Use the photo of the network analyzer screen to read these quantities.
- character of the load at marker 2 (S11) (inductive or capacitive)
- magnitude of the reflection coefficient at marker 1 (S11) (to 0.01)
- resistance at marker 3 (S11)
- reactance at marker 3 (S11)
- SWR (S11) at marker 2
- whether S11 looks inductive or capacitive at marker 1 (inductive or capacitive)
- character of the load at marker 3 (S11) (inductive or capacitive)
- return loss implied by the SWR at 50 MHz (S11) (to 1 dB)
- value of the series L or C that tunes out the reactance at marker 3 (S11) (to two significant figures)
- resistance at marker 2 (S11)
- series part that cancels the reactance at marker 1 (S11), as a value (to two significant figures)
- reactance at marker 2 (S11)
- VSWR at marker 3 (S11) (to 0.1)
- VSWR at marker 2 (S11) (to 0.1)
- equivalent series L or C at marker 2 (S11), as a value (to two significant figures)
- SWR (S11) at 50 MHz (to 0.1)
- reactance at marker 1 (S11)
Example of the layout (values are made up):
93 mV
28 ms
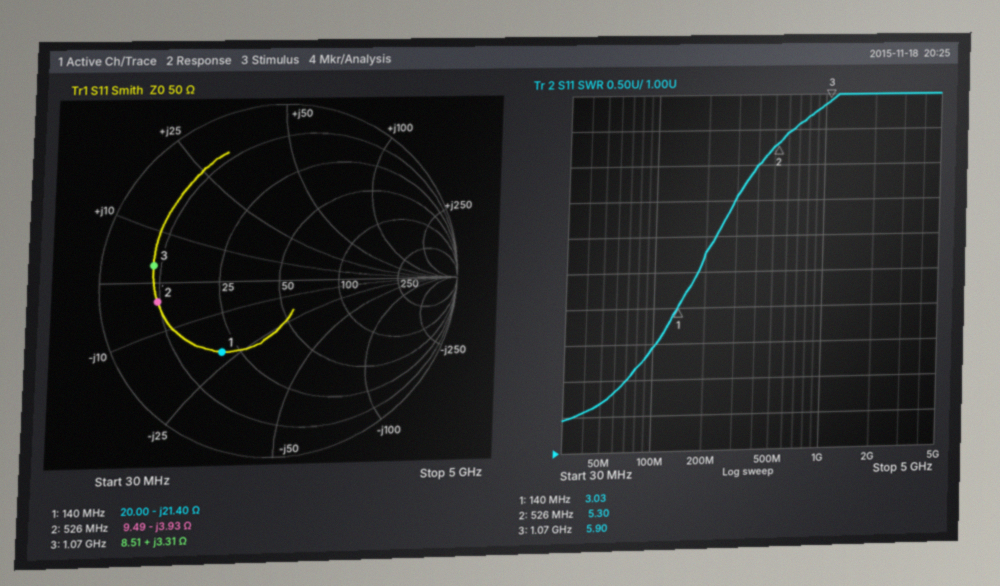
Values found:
capacitive
0.50
8.51 Ω
+3.31 Ω
5.30
capacitive
inductive
12 dB
45 pF
9.49 Ω
24 nH
-3.93 Ω
5.9
5.3
77 pF
1.7
-21.40 Ω
